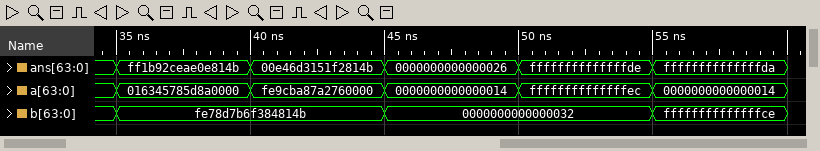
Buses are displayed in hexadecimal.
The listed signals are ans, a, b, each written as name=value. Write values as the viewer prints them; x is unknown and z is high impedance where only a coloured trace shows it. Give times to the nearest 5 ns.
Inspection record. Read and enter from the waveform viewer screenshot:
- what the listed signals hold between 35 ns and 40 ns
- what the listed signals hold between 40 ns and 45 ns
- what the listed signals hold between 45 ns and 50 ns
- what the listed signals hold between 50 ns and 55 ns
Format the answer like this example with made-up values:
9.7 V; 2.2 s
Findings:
ans=ff1b92ceae0e814b, a=016345785d8a0000, b=fe78d7b6f384814b; ans=00e46d3151f2814b, a=fe9cba87a2760000, b=fe78d7b6f384814b; ans=0000000000000026, a=0000000000000014, b=0000000000000032; ans=ffffffffffffffde, a=ffffffffffffffec, b=0000000000000032
